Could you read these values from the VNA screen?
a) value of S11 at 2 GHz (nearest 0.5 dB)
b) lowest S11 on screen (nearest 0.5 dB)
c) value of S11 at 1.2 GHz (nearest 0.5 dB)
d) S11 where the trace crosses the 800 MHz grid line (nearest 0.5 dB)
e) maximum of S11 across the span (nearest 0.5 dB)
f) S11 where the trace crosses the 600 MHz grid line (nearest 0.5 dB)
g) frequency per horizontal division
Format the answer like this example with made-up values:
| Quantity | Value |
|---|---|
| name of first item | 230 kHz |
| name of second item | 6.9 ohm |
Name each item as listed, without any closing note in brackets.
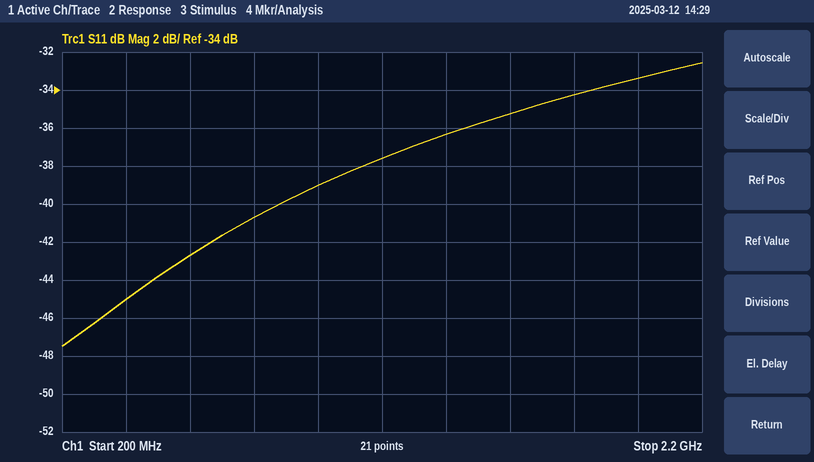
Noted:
| Quantity | Value |
|---|---|
| value of S11 at 2 GHz | -33.5 dB |
| lowest S11 on screen | -47.5 dB |
| value of S11 at 1.2 GHz | -37.5 dB |
| S11 where the trace crosses the 800 MHz grid line | -40.5 dB |
| maximum of S11 across the span | -32.5 dB |
| S11 where the trace crosses the 600 MHz grid line | -42.5 dB |
| frequency per horizontal division | 200 MHz |
